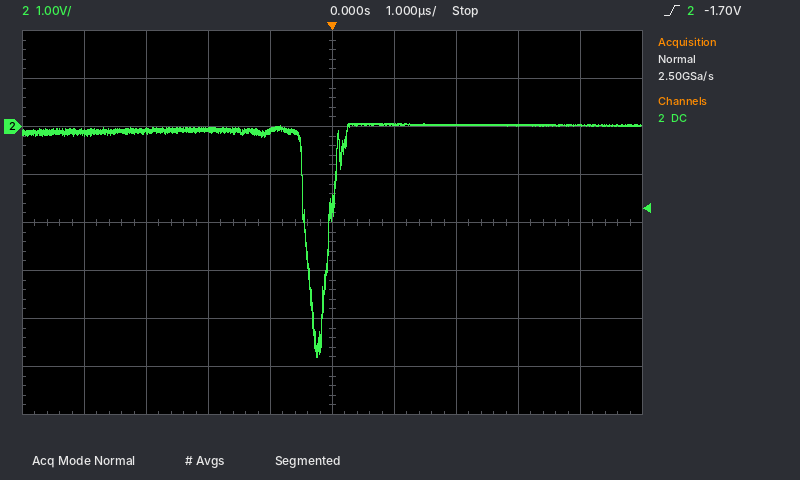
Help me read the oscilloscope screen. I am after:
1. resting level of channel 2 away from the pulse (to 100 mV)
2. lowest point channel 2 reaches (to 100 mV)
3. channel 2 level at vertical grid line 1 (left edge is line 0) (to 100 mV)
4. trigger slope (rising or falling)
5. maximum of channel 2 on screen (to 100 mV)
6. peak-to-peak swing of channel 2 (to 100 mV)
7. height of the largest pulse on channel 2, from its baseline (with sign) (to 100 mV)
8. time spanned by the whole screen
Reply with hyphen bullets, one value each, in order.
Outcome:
- 0.0 V
- -4.8 V
- -100 mV
- rising
- 100 mV
- 4.9 V
- -4.8 V
- 10 µs
